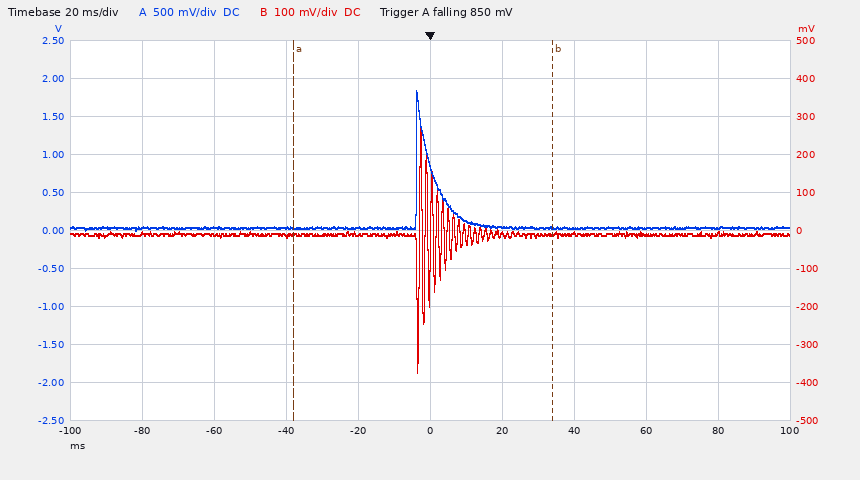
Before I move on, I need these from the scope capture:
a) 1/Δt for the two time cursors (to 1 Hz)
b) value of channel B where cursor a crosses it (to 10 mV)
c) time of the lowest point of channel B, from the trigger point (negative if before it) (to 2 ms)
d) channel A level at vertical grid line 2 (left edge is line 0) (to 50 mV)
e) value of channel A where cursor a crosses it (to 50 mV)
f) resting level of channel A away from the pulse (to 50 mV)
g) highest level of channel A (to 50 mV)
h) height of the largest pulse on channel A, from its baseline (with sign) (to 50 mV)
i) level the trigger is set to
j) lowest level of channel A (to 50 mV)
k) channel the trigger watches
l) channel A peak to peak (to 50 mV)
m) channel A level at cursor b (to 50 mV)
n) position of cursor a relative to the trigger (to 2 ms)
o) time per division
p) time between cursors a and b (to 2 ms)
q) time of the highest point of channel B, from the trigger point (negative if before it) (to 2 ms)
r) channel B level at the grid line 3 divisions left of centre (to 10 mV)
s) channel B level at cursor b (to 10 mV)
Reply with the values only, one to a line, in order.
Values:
14 Hz
-10 mV
-4 ms
50 mV
50 mV
50 mV
1.85 V
+1.80 V
850 mV
0 mV
channel A
1.85 V
50 mV
-38 ms
20 ms
72 ms
-2 ms
-10 mV
-10 mV
